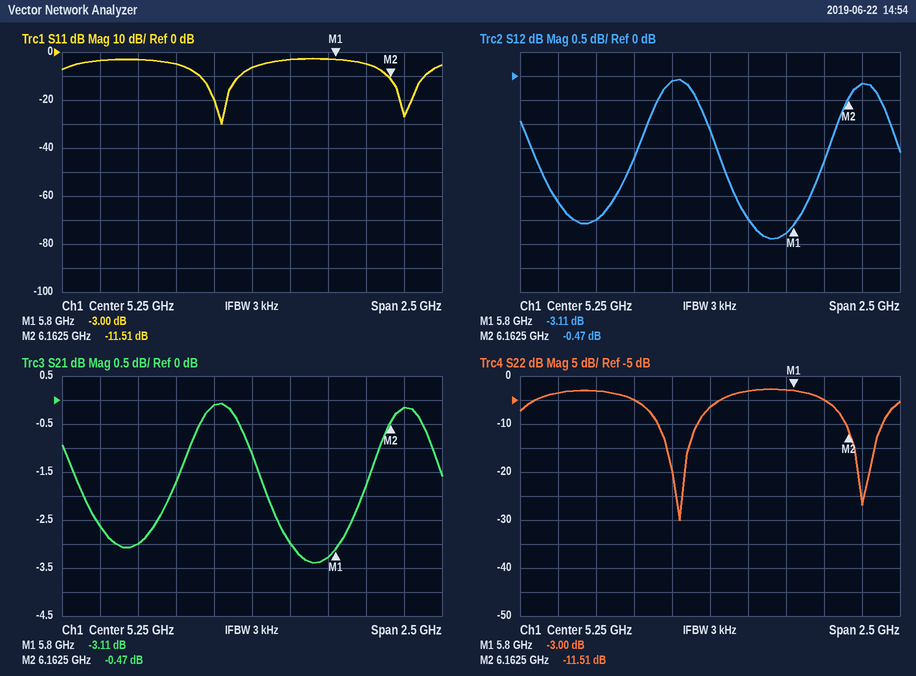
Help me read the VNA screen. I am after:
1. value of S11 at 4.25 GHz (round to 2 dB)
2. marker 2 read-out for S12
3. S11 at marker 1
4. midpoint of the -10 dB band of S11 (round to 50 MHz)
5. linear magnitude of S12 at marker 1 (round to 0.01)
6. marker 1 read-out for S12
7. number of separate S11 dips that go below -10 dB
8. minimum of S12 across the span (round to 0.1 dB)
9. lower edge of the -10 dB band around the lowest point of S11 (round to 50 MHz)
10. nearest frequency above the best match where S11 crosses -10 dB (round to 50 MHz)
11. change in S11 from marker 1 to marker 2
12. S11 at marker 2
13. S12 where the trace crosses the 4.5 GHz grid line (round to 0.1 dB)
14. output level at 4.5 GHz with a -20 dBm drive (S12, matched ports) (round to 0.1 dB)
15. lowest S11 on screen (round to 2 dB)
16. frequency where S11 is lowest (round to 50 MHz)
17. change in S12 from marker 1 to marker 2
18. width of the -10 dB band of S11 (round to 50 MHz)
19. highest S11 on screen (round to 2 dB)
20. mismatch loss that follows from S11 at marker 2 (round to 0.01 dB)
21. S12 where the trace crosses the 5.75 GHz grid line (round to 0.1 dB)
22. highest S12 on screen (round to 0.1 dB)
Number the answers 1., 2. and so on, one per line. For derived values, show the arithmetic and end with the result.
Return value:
1. -4 dB
2. -0.47 dB
3. -3.00 dB
4. 5.05 GHz
5. 10^(-3.11/20) ≈ 0.70
6. -3.11 dB
7. 2
8. -3.4 dB
9. 4.90 GHz
10. 5.15 GHz
11. -11.51 − (-3) = -8.51 dB
12. -11.51 dB
13. -3.0 dB
14. -20 dBm + (-3.0 dB) = -23.0 dBm
15. -30 dB
16. 5.05 GHz
17. -0.47 − (-3.11) = 2.64 dB
18. 5.15 GHz − 4.90 GHz = 250 MHz
19. -2 dB
20. −10 log10(1 − 10^(-11.51/10)) ≈ 0.32 dB
21. -3.3 dB
22. -0.1 dB
